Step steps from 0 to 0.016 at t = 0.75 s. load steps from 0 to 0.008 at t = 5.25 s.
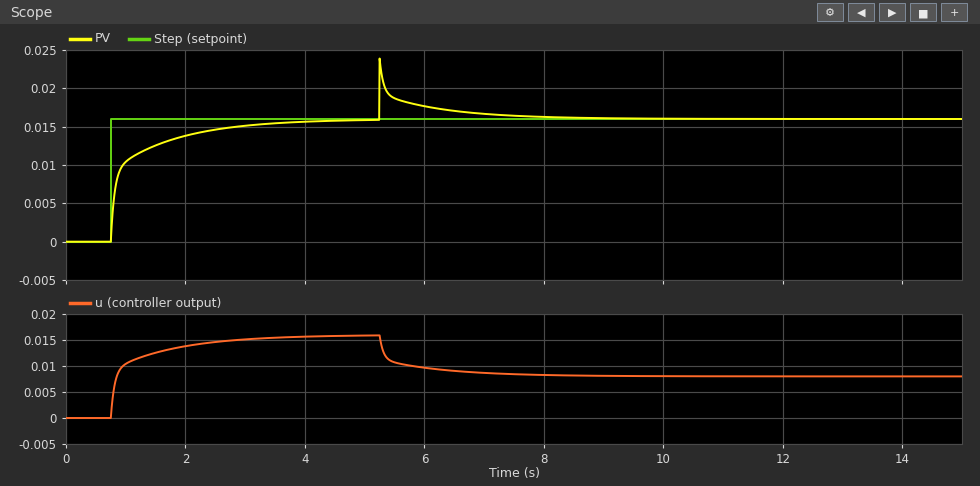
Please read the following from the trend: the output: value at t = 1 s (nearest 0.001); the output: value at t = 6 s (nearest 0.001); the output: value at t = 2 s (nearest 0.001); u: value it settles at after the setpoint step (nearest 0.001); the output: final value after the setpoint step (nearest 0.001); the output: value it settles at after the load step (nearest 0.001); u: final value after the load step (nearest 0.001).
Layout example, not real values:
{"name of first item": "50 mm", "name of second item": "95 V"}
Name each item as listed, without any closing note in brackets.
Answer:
{"the output: value at t = 1 s": "0.010", "the output: value at t = 6 s": "0.018", "the output: value at t = 2 s": "0.014", "u: value it settles at after the setpoint step": "0.016", "the output: final value after the setpoint step": "0.016", "the output: value it settles at after the load step": "0.016", "u: final value after the load step": "0.008"}
